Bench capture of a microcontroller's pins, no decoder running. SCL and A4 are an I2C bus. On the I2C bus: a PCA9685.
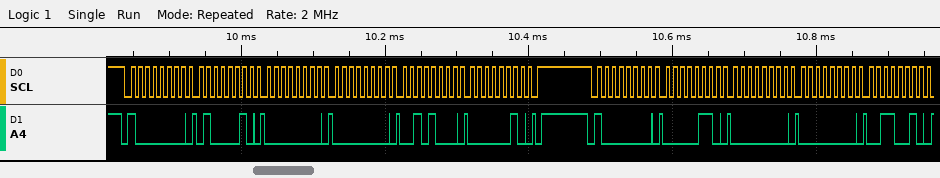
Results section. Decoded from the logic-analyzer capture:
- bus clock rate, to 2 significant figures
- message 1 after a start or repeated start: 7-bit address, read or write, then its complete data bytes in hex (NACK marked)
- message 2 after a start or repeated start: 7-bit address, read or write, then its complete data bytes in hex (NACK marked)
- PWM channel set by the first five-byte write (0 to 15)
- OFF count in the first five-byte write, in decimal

100 kHz
0x40 write: 42 00 00 28 02
0x40 write: 06 00 00 32
15
552
